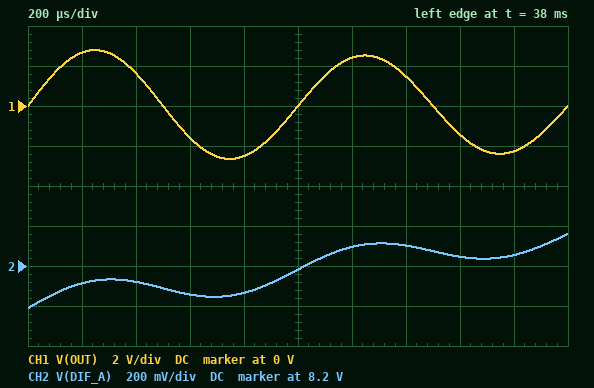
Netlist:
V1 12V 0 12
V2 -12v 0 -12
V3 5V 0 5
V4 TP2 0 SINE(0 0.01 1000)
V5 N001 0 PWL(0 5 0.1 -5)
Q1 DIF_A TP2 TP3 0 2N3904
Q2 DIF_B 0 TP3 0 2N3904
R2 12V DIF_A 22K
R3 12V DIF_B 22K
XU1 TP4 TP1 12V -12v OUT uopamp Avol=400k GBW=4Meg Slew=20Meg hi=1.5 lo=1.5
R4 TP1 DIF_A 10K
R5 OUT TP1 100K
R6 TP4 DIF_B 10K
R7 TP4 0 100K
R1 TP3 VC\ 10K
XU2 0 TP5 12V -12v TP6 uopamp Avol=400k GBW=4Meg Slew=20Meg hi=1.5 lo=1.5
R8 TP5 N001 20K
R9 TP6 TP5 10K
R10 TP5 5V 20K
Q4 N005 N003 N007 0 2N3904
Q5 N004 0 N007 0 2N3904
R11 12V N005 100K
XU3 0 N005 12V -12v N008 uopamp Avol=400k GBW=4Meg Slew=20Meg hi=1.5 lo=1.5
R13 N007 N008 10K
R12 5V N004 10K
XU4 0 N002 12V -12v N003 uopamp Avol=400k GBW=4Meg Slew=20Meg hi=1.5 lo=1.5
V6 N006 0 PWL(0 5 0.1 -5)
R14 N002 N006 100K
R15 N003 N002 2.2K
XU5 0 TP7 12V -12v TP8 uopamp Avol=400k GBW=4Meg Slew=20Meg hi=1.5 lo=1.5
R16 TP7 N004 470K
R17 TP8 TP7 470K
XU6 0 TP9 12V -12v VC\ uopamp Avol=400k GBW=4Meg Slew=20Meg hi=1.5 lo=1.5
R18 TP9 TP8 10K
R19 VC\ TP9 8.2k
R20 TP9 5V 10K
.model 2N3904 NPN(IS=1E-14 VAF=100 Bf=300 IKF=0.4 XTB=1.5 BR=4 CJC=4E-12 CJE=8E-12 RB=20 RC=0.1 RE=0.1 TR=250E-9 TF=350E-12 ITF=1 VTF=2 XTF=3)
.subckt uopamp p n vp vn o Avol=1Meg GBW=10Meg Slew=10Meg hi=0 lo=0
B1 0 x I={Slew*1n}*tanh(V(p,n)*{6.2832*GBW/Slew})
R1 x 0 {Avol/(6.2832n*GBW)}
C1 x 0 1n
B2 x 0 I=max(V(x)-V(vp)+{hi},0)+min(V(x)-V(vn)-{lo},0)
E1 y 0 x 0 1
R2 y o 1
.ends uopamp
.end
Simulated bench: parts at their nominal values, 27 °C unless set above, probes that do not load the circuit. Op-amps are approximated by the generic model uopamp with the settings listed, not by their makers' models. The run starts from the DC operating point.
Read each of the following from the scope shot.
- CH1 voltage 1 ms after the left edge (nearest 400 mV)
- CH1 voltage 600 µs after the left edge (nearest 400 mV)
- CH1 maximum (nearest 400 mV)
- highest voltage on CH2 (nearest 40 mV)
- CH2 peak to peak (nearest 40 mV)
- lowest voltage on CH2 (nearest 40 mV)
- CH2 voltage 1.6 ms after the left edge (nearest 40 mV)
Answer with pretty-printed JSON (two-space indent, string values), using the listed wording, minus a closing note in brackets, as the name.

{
  "CH1 voltage 1 ms after the left edge": "0 V",
  "CH1 voltage 600 µs after the left edge": "-1.6 V",
  "CH1 maximum": "2.8 V",
  "highest voltage on CH2": "8.36 V",
  "CH2 peak to peak": "360 mV",
  "lowest voltage on CH2": "8.00 V",
  "CH2 voltage 1.6 ms after the left edge": "8.24 V"
}
